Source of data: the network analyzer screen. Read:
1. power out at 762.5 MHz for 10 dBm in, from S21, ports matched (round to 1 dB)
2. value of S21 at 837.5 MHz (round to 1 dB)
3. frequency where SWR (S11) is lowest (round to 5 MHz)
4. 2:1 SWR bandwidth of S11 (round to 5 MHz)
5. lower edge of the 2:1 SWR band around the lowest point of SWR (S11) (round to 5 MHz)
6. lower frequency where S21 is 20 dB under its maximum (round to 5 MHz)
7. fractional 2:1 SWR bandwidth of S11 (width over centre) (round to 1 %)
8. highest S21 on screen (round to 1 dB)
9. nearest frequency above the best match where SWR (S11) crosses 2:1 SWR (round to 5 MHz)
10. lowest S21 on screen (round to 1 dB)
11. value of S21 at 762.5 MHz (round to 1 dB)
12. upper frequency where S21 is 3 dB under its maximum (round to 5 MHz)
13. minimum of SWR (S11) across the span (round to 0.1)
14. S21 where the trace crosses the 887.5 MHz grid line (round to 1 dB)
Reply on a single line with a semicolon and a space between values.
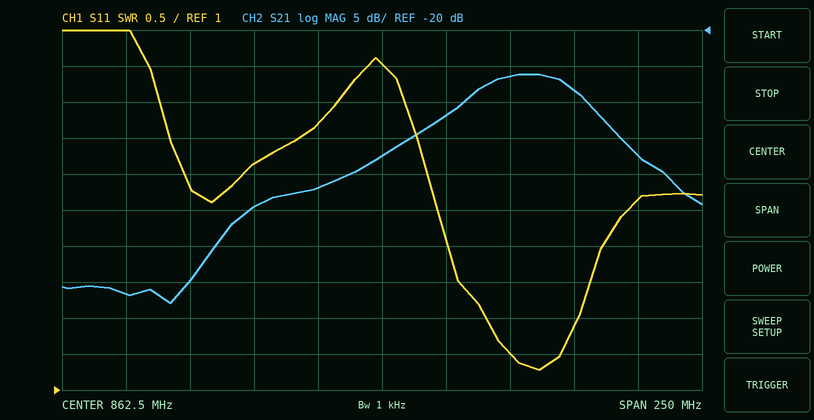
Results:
-47 dBm; -42 dB; 925 MHz; 35 MHz; 905 MHz; 805 MHz; 4 %; -26 dB; 940 MHz; -58 dB; -57 dB; 940 MHz; 1.3; -32 dB
